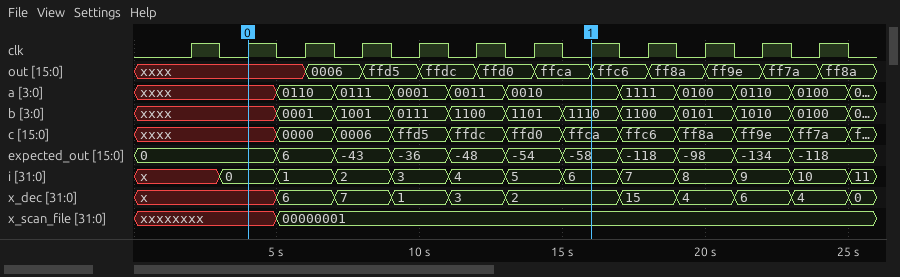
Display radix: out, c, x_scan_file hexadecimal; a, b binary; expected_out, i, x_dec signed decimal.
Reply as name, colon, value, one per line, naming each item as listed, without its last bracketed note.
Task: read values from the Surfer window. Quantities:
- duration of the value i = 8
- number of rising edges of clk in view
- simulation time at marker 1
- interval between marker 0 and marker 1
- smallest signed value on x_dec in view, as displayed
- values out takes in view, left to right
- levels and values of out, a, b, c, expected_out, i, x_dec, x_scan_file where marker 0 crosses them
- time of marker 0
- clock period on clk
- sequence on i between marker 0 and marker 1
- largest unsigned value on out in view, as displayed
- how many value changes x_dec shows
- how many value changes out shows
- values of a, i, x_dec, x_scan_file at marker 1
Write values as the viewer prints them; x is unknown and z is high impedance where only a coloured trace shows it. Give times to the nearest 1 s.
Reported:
duration of the value i = 8: 2 s
number of rising edges of clk in view: 12
simulation time at marker 1: 16 s
interval between marker 0 and marker 1: 12 s
smallest signed value on x_dec in view, as displayed: 0
values out takes in view, left to right: xxxx, 0006, ffd5, ffdc, ffd0, ffca, ffc6, ff8a, ff9e, ff7a, ff8a
levels and values of out, a, b, c, expected_out, i, x_dec, x_scan_file where marker 0 crosses them: out=xxxx, a=xxxx, b=xxxx, c=xxxx, expected_out=0, i=0, x_dec=x, x_scan_file=xxxxxxxx
time of marker 0: 4 s
clock period on clk: 2 s
sequence on i between marker 0 and marker 1: 0, 1, 2, 3, 4, 5, 6
largest unsigned value on out in view, as displayed: ffdc
how many value changes x_dec shows: 10
how many value changes out shows: 10
values of a, i, x_dec, x_scan_file at marker 1: a=0010, i=6, x_dec=2, x_scan_file=00000001
